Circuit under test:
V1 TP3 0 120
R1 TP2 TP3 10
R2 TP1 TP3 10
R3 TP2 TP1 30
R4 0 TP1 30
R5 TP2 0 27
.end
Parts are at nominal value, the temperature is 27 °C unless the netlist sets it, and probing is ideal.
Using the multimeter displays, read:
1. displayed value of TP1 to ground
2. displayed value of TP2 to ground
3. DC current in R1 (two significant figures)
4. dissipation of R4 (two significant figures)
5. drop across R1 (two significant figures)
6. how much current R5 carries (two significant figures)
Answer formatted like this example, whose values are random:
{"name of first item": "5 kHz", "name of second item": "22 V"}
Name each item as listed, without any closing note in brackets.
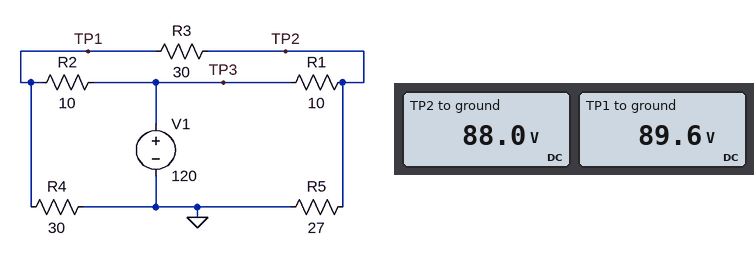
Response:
{"displayed value of TP1 to ground": "89.6 V", "displayed value of TP2 to ground": "88.0 V", "DC current in R1": "3.2 A", "dissipation of R4": "270 W", "drop across R1": "32 V", "how much current R5 carries": "3.3 A"}
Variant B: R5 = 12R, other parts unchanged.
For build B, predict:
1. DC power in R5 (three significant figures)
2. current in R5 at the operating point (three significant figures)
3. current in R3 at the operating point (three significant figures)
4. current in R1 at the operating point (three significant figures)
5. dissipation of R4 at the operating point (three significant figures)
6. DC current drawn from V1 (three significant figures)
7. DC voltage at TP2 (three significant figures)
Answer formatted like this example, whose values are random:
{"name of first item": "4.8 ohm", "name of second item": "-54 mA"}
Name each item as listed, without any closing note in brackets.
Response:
{"DC power in R5": "392 W", "current in R5 at the operating point": "5.71 A", "current in R3 at the operating point": "571 mA", "current in R1 at the operating point": "5.14 A", "dissipation of R4 at the operating point": "245 W", "DC current drawn from V1": "8.57 A", "DC voltage at TP2": "68.6 V"}
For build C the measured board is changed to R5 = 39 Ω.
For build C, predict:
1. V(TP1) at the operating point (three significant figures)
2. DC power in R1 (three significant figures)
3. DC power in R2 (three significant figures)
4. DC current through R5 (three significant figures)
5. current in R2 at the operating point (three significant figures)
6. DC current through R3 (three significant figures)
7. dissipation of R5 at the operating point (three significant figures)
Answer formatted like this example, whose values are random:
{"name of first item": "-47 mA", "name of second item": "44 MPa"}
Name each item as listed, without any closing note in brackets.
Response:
{"V(TP1) at the operating point": "90.9 V", "DC power in R1": "64.8 W", "DC power in R2": "84.6 W", "DC current through R5": "2.42 A", "current in R2 at the operating point": "2.91 A", "DC current through R3": "121 mA", "dissipation of R5 at the operating point": "229 W"}
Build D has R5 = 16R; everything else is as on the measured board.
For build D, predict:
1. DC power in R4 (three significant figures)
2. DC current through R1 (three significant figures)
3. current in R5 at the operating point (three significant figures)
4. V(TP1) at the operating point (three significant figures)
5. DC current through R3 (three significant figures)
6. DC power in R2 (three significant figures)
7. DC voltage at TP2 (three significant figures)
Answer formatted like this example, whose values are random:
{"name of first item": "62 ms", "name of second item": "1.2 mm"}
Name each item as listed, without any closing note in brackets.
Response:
{"DC power in R4": "254 W", "DC current through R1": "4.39 A", "current in R5 at the operating point": "4.76 A", "V(TP1) at the operating point": "87.2 V", "DC current through R3": "370 mA", "DC power in R2": "107 W", "DC voltage at TP2": "76.1 V"}
